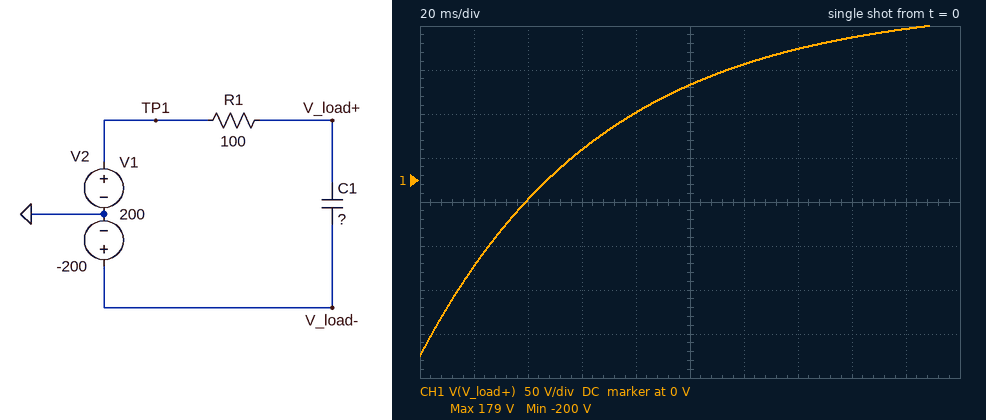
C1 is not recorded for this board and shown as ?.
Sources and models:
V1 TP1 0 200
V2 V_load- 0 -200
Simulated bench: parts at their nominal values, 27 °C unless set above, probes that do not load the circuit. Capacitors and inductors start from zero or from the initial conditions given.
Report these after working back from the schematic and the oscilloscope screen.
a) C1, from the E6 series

680 µF
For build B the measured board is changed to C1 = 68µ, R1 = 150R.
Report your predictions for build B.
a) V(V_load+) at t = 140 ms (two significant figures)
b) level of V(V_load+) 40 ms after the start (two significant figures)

200 V
190 V
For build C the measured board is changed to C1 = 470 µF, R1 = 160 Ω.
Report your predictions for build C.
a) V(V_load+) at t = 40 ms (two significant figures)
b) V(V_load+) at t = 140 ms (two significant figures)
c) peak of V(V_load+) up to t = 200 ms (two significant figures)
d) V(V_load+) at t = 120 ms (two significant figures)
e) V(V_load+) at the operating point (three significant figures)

-35 V
140 V
170 V
120 V
200 V
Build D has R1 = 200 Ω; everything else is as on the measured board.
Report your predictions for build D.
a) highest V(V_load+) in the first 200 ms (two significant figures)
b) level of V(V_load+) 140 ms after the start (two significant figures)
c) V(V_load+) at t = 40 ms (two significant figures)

110 V
57 V
-98 V
